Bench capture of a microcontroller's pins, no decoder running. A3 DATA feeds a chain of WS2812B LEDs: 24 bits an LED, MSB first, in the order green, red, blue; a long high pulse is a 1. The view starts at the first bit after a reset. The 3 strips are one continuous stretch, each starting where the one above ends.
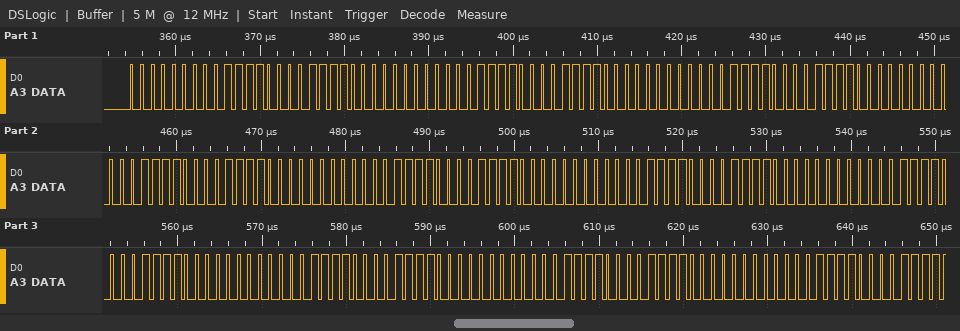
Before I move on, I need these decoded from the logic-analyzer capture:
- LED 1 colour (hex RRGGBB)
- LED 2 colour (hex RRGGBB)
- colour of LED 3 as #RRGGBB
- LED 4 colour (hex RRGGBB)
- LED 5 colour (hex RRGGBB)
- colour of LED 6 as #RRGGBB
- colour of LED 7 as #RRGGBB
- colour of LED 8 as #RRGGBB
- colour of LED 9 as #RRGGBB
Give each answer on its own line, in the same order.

#780078
#780078
#780078
#780078
#780078
#780078
#780078
#780078
#780078
